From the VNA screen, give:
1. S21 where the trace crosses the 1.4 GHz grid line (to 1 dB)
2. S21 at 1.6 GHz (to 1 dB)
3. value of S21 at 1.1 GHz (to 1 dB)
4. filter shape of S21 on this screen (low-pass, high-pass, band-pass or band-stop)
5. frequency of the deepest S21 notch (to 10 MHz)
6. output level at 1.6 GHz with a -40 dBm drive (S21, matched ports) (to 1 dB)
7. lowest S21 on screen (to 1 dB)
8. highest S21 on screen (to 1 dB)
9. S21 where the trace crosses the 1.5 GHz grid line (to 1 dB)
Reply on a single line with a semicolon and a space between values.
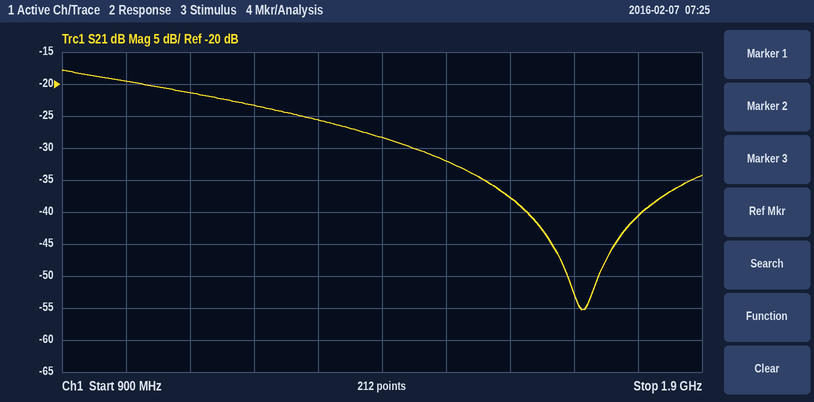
-28 dB; -38 dB; -21 dB; low-pass; 1.71 GHz; -78 dBm; -55 dB; -18 dB; -32 dB
